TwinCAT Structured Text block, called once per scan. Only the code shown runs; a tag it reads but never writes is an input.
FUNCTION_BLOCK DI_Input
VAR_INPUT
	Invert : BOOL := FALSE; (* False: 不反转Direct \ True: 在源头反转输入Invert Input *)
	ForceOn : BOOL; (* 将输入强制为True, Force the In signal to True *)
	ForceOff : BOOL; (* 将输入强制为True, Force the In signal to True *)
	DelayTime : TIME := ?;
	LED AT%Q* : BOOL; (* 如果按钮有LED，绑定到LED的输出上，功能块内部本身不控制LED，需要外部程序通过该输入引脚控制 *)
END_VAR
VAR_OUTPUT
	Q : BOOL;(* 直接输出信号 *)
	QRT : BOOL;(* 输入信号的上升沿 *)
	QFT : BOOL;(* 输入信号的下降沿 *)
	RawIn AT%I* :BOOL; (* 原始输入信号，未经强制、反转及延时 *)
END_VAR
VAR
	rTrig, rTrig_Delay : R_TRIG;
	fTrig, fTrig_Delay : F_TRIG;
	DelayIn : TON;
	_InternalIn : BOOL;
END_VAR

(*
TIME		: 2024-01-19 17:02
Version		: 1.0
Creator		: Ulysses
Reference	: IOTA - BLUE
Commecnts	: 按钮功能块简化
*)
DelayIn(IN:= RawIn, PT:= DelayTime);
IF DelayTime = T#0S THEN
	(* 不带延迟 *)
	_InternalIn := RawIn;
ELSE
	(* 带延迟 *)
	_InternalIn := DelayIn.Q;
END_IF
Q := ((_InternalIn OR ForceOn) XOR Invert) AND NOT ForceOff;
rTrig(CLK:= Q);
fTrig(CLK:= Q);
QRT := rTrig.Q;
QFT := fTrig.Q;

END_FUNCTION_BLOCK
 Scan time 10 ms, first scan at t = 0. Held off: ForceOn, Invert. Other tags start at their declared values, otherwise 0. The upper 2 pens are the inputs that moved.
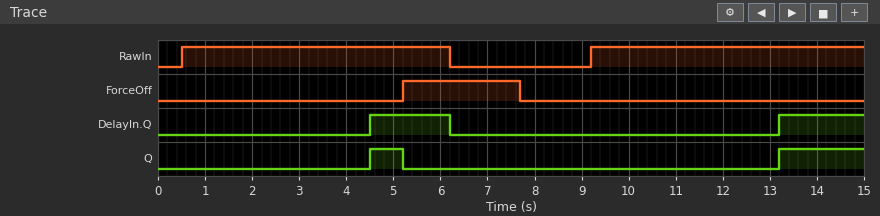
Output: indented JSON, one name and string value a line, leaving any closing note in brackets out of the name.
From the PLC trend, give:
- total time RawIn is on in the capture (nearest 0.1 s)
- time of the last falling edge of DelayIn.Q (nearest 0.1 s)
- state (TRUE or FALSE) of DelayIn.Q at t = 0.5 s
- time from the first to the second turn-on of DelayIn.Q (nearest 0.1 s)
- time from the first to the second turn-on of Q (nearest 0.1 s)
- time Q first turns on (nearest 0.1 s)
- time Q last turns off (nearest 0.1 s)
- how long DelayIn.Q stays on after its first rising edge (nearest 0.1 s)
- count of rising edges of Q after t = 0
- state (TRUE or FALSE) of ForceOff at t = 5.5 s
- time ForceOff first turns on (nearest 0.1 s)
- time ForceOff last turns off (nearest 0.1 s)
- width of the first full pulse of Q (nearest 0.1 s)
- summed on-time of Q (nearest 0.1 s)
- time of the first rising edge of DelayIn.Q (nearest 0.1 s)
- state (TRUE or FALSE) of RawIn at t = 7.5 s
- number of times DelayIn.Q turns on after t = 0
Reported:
{
  "total time RawIn is on in the capture": "11.5 s",
  "time of the last falling edge of DelayIn.Q": "6.2 s",
  "state (TRUE or FALSE) of DelayIn.Q at t = 0.5 s": "FALSE",
  "time from the first to the second turn-on of DelayIn.Q": "8.7 s",
  "time from the first to the second turn-on of Q": "8.7 s",
  "time Q first turns on": "4.5 s",
  "time Q last turns off": "5.2 s",
  "how long DelayIn.Q stays on after its first rising edge": "1.7 s",
  "count of rising edges of Q after t = 0": "2",
  "state (TRUE or FALSE) of ForceOff at t = 5.5 s": "TRUE",
  "time ForceOff first turns on": "5.2 s",
  "time ForceOff last turns off": "7.7 s",
  "width of the first full pulse of Q": "0.7 s",
  "summed on-time of Q": "2.5 s",
  "time of the first rising edge of DelayIn.Q": "4.5 s",
  "state (TRUE or FALSE) of RawIn at t = 7.5 s": "FALSE",
  "number of times DelayIn.Q turns on after t = 0": "2"
}
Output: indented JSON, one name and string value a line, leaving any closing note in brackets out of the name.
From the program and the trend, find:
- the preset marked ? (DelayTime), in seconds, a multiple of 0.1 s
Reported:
{
  "the preset marked ? (DelayTime), in seconds, a multiple of 0.1 s": "4.0 s"
}
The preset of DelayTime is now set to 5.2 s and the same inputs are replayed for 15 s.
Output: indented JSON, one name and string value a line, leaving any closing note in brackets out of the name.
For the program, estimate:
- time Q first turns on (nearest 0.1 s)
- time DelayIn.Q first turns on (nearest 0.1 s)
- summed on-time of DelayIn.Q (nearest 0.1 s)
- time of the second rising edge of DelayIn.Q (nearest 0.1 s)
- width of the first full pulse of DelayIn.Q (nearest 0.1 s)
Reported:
{
  "time Q first turns on": "14.4 s",
  "time DelayIn.Q first turns on": "5.7 s",
  "summed on-time of DelayIn.Q": "1.1 s",
  "time of the second rising edge of DelayIn.Q": "14.4 s",
  "width of the first full pulse of DelayIn.Q": "0.5 s"
}
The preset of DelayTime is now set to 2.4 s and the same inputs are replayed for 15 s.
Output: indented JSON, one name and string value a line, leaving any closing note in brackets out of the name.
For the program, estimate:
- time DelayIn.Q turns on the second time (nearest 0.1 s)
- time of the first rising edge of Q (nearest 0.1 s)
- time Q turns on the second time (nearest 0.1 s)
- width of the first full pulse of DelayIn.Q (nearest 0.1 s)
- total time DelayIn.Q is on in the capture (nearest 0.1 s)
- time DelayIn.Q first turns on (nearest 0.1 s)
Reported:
{
  "time DelayIn.Q turns on the second time": "11.6 s",
  "time of the first rising edge of Q": "2.9 s",
  "time Q turns on the second time": "11.6 s",
  "width of the first full pulse of DelayIn.Q": "3.3 s",
  "total time DelayIn.Q is on in the capture": "6.7 s",
  "time DelayIn.Q first turns on": "2.9 s"
}
